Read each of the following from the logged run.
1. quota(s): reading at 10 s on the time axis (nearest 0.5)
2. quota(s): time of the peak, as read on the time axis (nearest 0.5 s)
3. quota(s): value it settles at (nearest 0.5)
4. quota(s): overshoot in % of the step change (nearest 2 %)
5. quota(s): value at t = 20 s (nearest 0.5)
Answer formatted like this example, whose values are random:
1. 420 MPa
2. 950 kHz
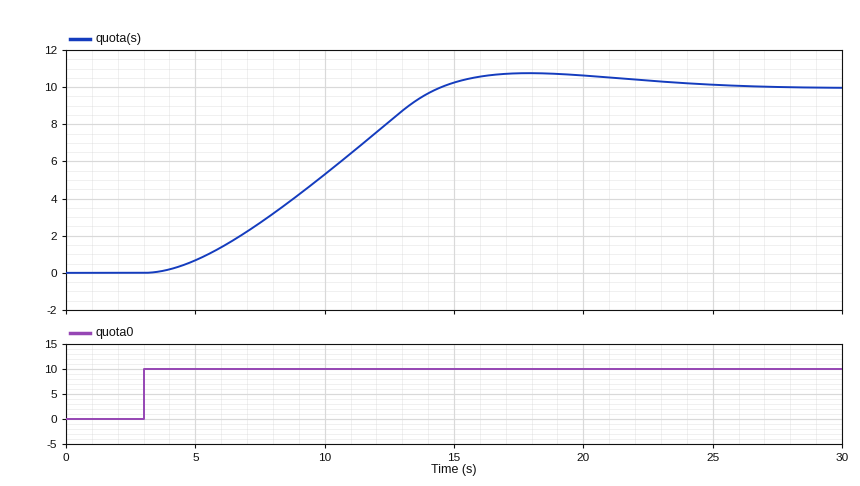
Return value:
1. 5.5
2. 18.0 s
3. 10.0
4. 8 %
5. 10.5
